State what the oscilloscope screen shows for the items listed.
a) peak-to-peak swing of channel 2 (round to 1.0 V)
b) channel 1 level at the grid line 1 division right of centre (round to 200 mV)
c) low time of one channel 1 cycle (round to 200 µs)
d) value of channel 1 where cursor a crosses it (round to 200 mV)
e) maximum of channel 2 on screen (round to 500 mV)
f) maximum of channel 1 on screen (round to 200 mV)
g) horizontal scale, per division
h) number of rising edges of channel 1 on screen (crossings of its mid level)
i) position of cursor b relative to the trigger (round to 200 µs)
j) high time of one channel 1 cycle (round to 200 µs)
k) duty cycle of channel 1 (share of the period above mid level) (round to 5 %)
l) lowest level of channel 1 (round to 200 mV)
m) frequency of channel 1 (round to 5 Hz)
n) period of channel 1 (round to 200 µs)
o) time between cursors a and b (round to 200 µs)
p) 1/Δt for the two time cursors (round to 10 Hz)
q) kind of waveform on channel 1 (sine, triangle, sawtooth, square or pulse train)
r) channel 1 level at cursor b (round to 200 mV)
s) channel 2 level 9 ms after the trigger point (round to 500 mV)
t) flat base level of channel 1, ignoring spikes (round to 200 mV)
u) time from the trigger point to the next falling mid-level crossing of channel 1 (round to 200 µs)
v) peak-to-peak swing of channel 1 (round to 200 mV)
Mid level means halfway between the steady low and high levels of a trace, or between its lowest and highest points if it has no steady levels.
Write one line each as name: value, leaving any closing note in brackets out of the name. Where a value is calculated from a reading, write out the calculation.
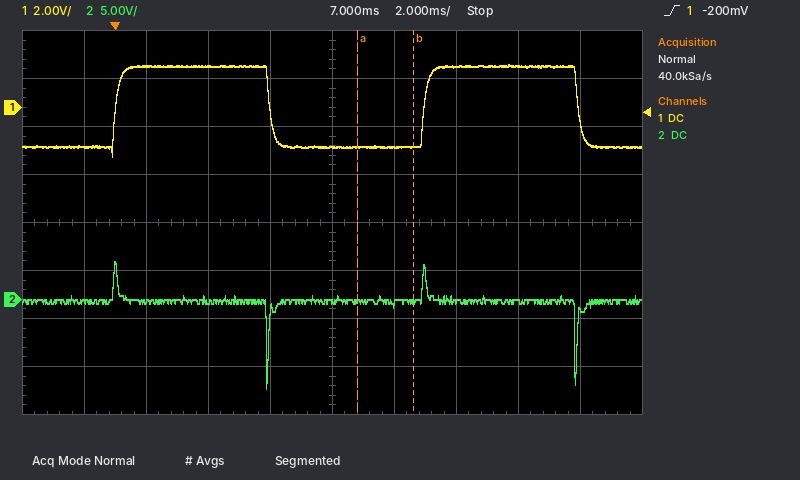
peak-to-peak swing of channel 2: 13.0 V
channel 1 level at the grid line 1 division right of centre: -1.6 V
low time of one channel 1 cycle: 5.0 ms
value of channel 1 where cursor a crosses it: -1.6 V
maximum of channel 2 on screen: 4.0 V
maximum of channel 1 on screen: 1.8 V
horizontal scale, per division: 2 ms
number of rising edges of channel 1 on screen: 2
position of cursor b relative to the trigger: +9.6 ms
high time of one channel 1 cycle: 5.0 ms
duty cycle of channel 1 (share of the period above mid level): 5.0 ms / 10.0 ms ≈ 50 %
lowest level of channel 1: -2.0 V
frequency of channel 1: 1 / 10.0 ms ≈ 100 Hz
period of channel 1: 10.0 ms
time between cursors a and b: 1.8 ms
1/Δt for the two time cursors: 1 / 1.8 ms ≈ 560 Hz
kind of waveform on channel 1: square
channel 1 level at cursor b: -1.6 V
channel 2 level 9 ms after the trigger point: -500 mV
flat base level of channel 1, ignoring spikes: -1.6 V
time from the trigger point to the next falling mid-level crossing of channel 1: 5.0 ms
peak-to-peak swing of channel 1: 1.8 V − (-2.0 V) = 3.8 V
